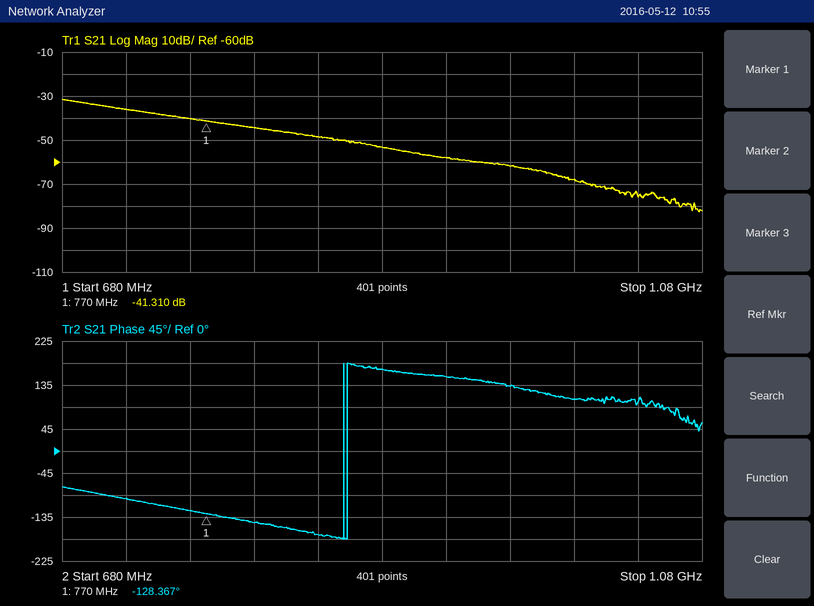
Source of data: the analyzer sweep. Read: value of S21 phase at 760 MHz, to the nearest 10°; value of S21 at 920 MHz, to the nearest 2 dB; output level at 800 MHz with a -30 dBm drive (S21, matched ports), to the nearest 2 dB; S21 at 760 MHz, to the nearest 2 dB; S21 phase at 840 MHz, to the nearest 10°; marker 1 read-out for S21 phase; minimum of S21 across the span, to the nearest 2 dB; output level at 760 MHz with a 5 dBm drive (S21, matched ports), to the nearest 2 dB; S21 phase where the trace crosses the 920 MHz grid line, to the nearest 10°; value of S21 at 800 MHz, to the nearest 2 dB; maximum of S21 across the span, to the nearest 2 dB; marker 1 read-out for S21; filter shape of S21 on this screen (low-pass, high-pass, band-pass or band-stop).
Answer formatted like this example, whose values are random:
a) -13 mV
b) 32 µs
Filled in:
a) -120°
b) -58 dB
c) -74 dBm
d) -40 dB
e) -170°
f) -128.367°
g) -82 dB
h) -36 dBm
i) 150°
j) -44 dB
k) -32 dB
l) -41.310 dB
m) low-pass
